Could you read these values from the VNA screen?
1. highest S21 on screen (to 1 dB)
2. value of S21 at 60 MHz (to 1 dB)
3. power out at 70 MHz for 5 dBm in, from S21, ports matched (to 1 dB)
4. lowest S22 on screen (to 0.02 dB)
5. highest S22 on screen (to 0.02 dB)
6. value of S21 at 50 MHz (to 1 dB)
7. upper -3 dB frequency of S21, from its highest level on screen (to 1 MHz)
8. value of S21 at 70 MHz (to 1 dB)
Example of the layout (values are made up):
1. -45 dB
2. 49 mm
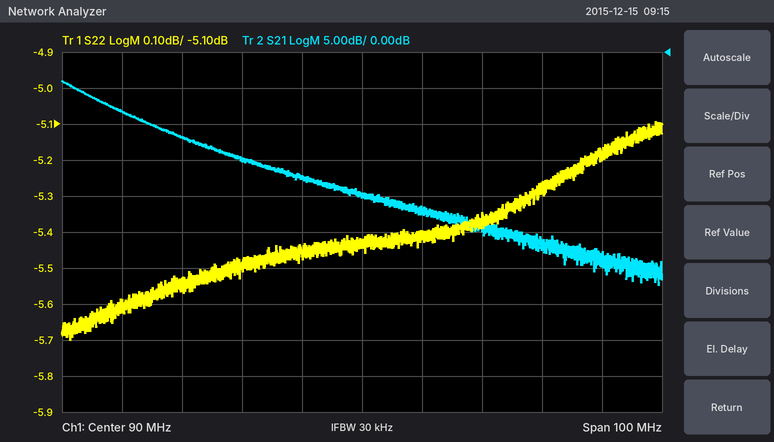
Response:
1. -4 dB
2. -12 dB
3. -10 dBm
4. -5.70 dB
5. -5.10 dB
6. -8 dB
7. 47 MHz
8. -15 dB
